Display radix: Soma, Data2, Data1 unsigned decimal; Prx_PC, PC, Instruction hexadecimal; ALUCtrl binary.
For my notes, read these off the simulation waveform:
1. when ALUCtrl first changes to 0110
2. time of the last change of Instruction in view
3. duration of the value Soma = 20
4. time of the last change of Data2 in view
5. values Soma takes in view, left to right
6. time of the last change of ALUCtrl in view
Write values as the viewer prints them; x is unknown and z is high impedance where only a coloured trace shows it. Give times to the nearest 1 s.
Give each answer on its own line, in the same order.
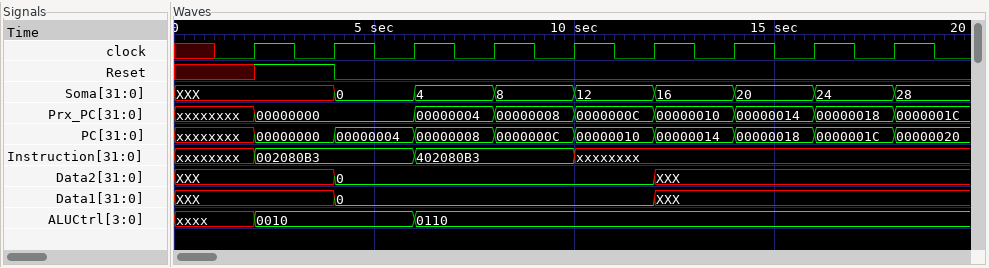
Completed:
6 s
10 s
2 s
12 s
XXX, 0, 4, 8, 12, 16, 20, 24, 28
6 s
